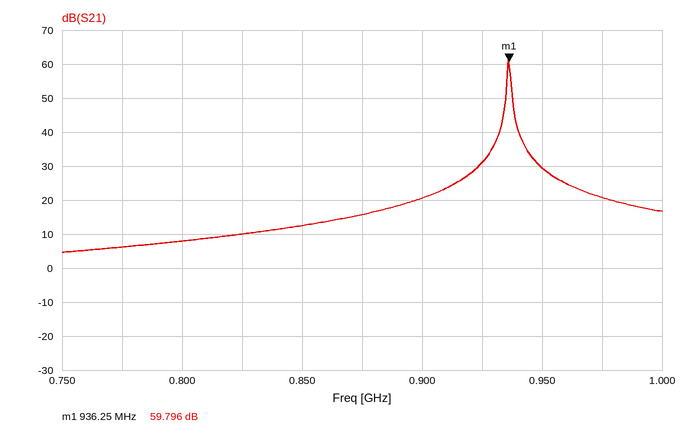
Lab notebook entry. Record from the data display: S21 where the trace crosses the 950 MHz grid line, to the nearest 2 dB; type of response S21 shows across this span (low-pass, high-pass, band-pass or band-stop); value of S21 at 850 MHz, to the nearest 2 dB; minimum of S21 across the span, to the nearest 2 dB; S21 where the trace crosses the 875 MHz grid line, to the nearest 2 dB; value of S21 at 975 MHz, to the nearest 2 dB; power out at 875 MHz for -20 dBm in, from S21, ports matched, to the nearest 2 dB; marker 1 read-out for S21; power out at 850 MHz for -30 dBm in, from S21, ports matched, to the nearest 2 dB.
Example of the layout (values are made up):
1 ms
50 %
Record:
30 dB
band-pass
12 dB
4 dB
16 dB
20 dB
-4 dBm
59.796 dB
-18 dBm
